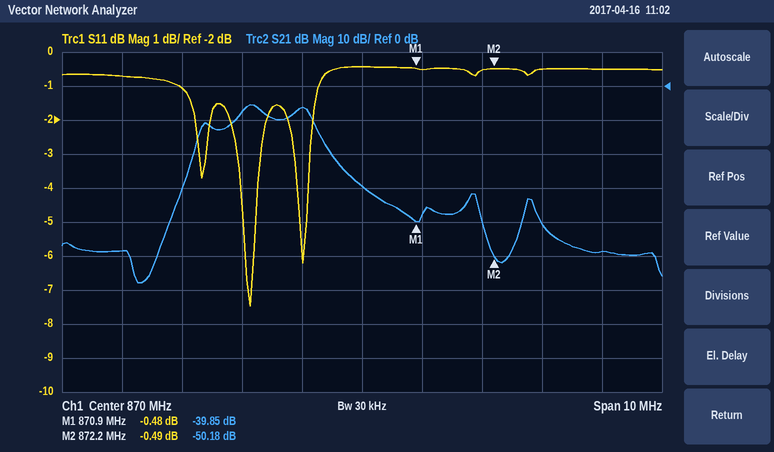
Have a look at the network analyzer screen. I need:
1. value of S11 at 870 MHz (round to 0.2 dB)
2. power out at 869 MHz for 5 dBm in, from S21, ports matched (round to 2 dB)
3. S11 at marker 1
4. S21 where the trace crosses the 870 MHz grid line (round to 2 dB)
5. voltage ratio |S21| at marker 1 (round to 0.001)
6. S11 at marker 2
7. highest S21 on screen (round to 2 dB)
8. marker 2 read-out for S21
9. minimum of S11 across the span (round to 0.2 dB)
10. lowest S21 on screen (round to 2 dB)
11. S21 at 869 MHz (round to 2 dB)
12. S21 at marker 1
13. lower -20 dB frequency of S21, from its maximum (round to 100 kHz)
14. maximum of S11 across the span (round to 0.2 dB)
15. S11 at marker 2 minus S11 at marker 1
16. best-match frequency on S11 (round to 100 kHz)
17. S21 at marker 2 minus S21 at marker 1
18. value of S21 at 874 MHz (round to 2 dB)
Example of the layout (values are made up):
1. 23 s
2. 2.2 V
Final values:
1. -0.4 dB
2. -2 dBm
3. -0.48 dB
4. -30 dB
5. 0.010
6. -0.49 dB
7. -6 dB
8. -50.18 dB
9. -7.4 dB
10. -58 dB
11. -6 dB
12. -39.85 dB
13. 867.1 MHz
14. -0.4 dB
15. -0.01 dB
16. 868.1 MHz
17. -10.33 dB
18. -48 dB
